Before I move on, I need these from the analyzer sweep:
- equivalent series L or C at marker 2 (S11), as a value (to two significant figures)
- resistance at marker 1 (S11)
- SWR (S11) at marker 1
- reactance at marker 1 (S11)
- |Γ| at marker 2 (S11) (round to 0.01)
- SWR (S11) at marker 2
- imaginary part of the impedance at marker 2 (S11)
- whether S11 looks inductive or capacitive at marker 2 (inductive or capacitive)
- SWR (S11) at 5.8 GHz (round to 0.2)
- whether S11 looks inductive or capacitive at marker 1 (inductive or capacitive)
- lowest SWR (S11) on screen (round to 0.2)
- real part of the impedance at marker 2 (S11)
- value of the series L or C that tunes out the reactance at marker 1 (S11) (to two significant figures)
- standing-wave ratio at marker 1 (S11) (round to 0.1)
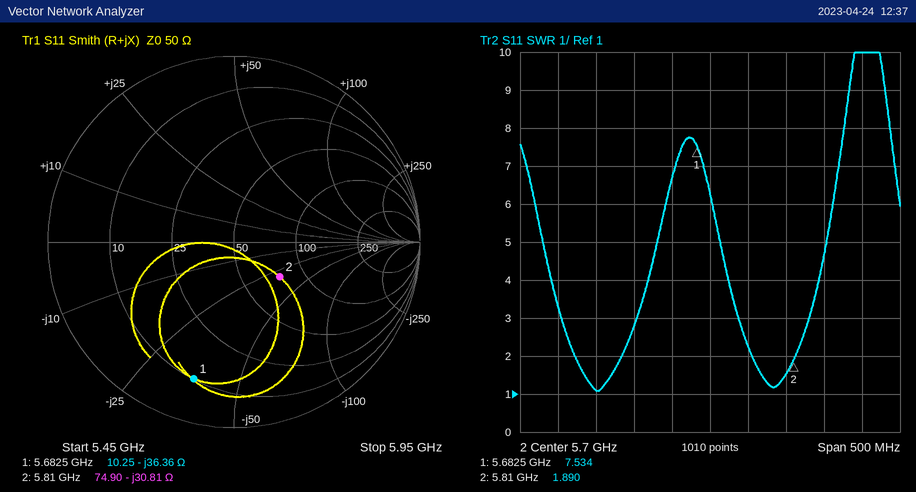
890 fF
10.25 Ω
7.534
-36.36 Ω
0.31
1.890
-30.81 Ω
capacitive
1.6
capacitive
1.0
74.90 Ω
1.0 nH
7.5
